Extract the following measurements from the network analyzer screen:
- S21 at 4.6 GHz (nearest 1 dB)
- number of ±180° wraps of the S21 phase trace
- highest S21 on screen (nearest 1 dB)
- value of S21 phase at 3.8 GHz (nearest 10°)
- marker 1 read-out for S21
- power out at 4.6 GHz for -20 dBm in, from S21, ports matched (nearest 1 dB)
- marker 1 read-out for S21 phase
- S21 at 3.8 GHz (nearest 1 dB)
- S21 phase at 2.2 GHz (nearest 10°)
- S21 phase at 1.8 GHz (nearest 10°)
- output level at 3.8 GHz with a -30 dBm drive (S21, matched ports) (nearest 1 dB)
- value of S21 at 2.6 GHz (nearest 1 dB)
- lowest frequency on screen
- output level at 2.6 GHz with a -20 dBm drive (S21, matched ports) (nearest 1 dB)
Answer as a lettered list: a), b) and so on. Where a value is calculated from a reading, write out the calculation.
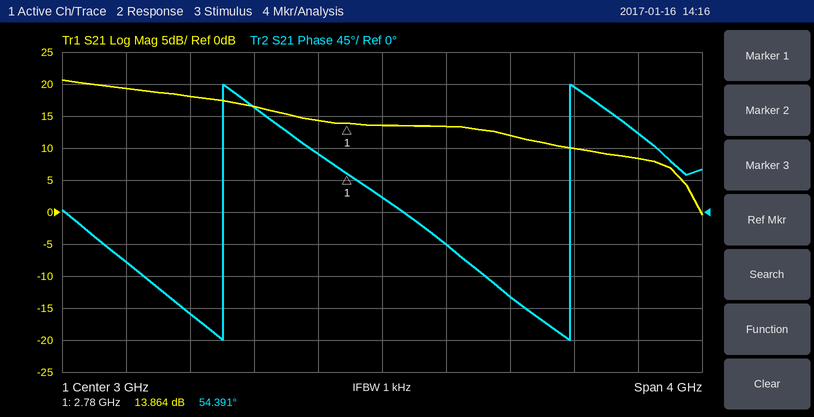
a) 8 dB
b) 2
c) 21 dB
d) -120°
e) 13.864 dB
f) -20 dBm + (8 dB) = -12 dBm
g) 54.391°
h) 12 dB
i) 150°
j) -140°
k) -30 dBm + (12 dB) = -18 dBm
l) 14 dB
m) 1 GHz
n) -20 dBm + (14 dB) = -6 dBm
